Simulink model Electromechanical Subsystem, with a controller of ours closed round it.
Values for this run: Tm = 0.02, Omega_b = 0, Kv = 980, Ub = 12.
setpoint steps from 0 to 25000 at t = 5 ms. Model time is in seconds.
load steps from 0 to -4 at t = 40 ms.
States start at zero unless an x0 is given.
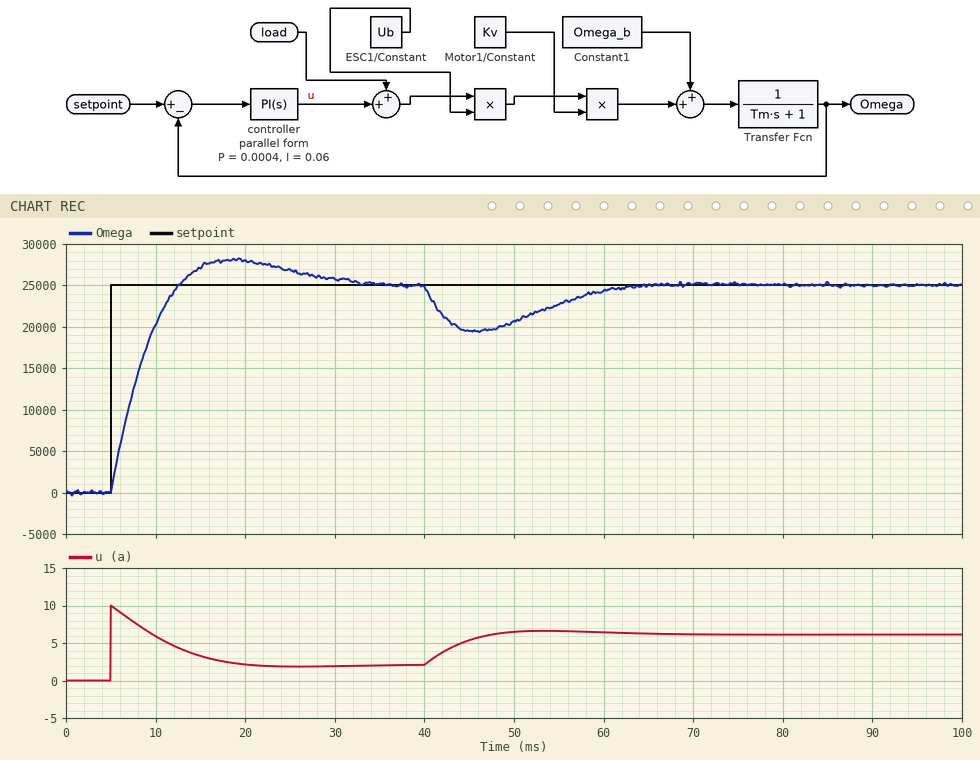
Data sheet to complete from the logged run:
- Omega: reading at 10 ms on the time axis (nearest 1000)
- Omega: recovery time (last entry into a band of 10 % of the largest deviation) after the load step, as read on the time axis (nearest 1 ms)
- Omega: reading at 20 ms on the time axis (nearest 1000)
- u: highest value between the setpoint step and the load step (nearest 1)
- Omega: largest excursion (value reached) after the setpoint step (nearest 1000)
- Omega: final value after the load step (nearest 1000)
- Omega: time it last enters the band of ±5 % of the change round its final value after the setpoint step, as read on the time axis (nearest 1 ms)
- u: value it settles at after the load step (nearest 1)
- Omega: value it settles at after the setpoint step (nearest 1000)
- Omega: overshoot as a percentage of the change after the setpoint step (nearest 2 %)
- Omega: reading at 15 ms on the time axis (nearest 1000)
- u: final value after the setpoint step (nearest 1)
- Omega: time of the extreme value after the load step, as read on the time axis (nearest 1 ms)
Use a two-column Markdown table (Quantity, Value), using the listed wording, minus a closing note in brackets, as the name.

| Quantity | Value |
|---|---|
| Omega: reading at 10 ms on the time axis | 20000 |
| Omega: recovery time (last entry into a band of 10 % of the largest deviation) after the load step, as read on the time axis | 61 ms |
| Omega: reading at 20 ms on the time axis | 28000 |
| u: highest value between the setpoint step and the load step | 10 |
| Omega: largest excursion (value reached) after the setpoint step | 28000 |
| Omega: final value after the load step | 25000 |
| Omega: time it last enters the band of ±5 % of the change round its final value after the setpoint step, as read on the time axis | 27 ms |
| u: value it settles at after the load step | 6 |
| Omega: value it settles at after the setpoint step | 25000 |
| Omega: overshoot as a percentage of the change after the setpoint step | 12 % |
| Omega: reading at 15 ms on the time axis | 27000 |
| u: final value after the setpoint step | 2 |
| Omega: time of the extreme value after the load step, as read on the time axis | 46 ms |
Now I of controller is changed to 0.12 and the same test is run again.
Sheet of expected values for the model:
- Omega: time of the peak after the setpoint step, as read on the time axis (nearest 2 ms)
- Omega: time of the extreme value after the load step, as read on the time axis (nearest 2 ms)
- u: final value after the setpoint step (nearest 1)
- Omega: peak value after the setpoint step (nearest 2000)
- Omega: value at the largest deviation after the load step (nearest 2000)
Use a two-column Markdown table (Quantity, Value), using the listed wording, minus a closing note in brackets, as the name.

| Quantity | Value |
|---|---|
| Omega: time of the peak after the setpoint step, as read on the time axis | 14 ms |
| Omega: time of the extreme value after the load step, as read on the time axis | 44 ms |
| u: final value after the setpoint step | 2 |
| Omega: peak value after the setpoint step | 30000 |
| Omega: value at the largest deviation after the load step | 20000 |
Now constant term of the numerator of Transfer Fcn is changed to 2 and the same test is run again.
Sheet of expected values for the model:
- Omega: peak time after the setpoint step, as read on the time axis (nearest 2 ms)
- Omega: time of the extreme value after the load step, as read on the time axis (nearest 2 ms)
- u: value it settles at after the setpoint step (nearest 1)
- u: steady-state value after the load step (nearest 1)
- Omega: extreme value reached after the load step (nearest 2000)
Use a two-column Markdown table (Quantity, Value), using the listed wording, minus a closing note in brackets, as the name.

| Quantity | Value |
|---|---|
| Omega: peak time after the setpoint step, as read on the time axis | 14 ms |
| Omega: time of the extreme value after the load step, as read on the time axis | 44 ms |
| u: value it settles at after the setpoint step | 1 |
| u: steady-state value after the load step | 5 |
| Omega: extreme value reached after the load step | 18000 |
